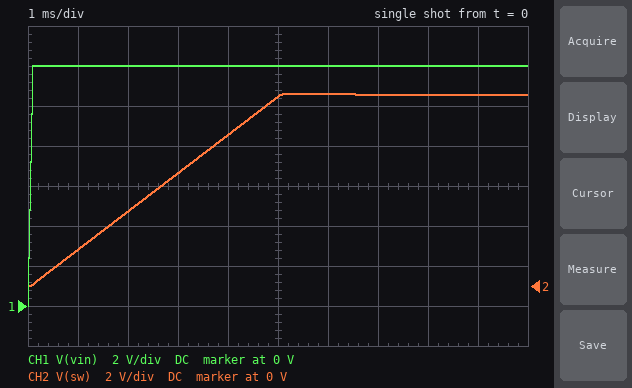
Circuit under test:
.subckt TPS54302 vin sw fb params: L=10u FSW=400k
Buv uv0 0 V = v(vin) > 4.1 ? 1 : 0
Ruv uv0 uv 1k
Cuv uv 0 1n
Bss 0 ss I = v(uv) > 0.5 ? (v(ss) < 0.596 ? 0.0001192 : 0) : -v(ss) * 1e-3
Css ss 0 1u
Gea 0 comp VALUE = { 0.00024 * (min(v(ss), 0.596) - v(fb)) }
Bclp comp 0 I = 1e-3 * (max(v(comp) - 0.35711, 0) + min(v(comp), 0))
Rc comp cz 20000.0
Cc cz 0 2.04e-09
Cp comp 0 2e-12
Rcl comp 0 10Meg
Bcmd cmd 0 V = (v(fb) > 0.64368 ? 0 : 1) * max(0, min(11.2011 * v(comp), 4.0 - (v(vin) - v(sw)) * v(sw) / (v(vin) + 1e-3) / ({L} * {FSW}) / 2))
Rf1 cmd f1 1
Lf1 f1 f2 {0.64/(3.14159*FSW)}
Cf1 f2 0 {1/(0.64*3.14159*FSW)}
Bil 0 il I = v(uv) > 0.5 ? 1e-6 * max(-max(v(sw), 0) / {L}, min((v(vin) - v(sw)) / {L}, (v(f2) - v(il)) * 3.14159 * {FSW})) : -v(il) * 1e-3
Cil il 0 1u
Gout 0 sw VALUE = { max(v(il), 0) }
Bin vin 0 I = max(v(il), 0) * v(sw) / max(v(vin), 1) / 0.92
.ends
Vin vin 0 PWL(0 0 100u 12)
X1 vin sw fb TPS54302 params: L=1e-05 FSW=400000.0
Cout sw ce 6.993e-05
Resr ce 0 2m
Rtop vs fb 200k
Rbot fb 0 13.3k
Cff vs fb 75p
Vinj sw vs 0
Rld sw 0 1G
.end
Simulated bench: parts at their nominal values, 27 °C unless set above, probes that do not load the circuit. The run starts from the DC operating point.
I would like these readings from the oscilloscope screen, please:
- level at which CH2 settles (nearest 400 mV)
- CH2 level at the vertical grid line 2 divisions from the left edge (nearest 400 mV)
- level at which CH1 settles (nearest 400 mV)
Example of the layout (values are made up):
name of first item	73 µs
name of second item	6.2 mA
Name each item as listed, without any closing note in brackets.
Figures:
level at which CH2 settles	9.6 V
CH2 level at the vertical grid line 2 divisions from the left edge	3.6 V
level at which CH1 settles	12.0 V
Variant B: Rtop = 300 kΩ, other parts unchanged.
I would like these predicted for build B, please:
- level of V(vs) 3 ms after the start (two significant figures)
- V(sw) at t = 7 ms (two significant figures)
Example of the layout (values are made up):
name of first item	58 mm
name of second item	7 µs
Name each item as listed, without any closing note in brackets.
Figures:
level of V(vs) 3 ms after the start	8.3 V
V(sw) at t = 7 ms	12 V
